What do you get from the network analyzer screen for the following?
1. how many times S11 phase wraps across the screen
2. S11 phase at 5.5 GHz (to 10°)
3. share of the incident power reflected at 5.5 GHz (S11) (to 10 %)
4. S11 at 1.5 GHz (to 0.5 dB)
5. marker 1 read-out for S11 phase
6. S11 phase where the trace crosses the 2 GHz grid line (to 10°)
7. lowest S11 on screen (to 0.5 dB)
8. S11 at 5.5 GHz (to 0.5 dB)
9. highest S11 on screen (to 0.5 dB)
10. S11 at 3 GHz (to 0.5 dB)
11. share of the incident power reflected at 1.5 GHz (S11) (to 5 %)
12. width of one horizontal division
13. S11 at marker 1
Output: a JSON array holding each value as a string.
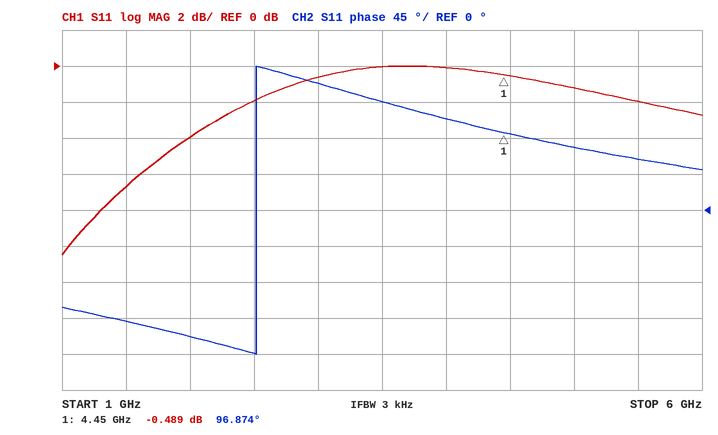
["1", "60°", "60 %", "-6.5 dB", "96.874°", "-160°", "-10.5 dB", "-2.0 dB", "0.0 dB", "-0.5 dB", "20 %", "500 MHz", "-0.489 dB"]
